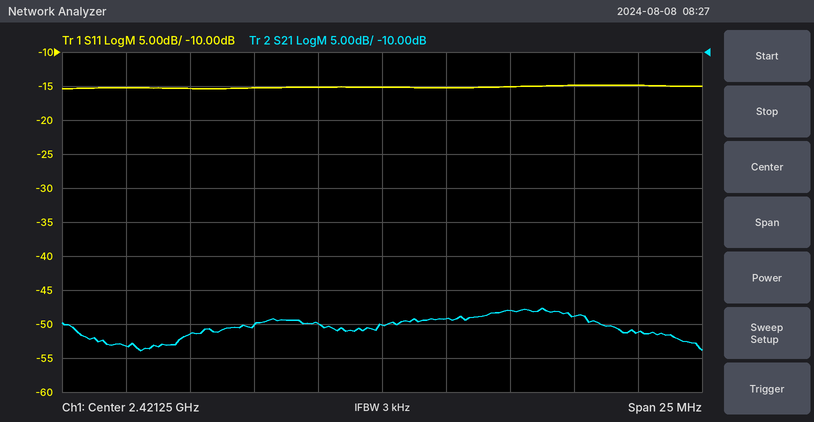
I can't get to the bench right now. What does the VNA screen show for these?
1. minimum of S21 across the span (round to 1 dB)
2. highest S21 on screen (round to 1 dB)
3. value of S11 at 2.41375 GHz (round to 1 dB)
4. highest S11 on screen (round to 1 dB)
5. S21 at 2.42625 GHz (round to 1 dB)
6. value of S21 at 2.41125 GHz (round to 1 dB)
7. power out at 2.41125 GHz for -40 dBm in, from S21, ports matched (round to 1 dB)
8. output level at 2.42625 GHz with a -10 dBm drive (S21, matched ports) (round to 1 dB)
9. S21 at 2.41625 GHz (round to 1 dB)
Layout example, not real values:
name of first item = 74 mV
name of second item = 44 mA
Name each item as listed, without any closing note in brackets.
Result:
minimum of S21 across the span = -54 dB
highest S21 on screen = -48 dB
value of S11 at 2.41375 GHz = -15 dB
highest S11 on screen = -15 dB
S21 at 2.42625 GHz = -48 dB
value of S21 at 2.41125 GHz = -53 dB
power out at 2.41125 GHz for -40 dBm in, from S21, ports matched = -93 dBm
output level at 2.42625 GHz with a -10 dBm drive (S21, matched ports) = -58 dBm
S21 at 2.41625 GHz = -50 dB
